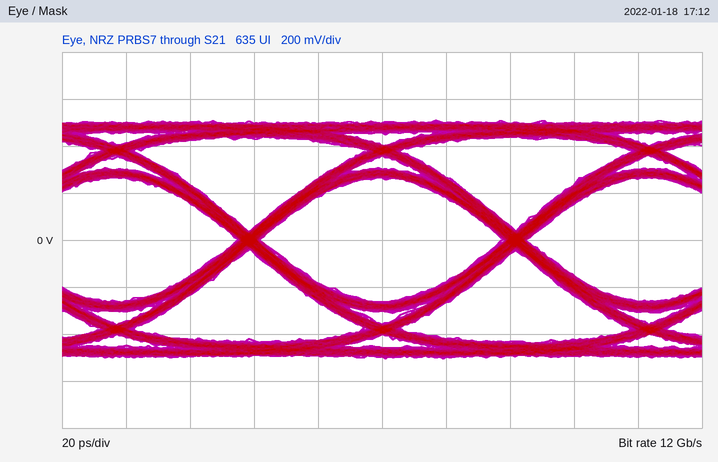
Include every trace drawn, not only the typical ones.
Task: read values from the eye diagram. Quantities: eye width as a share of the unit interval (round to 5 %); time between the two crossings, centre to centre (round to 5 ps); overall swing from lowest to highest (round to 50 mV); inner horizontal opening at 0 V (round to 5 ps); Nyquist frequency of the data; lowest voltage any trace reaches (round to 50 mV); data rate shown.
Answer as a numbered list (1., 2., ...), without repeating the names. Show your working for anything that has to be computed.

1. 75 ps / 85 ps ≈ 88.2 %, so 90 % to the nearest 5 %
2. 85 ps
3. 1.00 V
4. 75 ps
5. 6 GHz
6. -500 mV
7. 12 Gb/s
